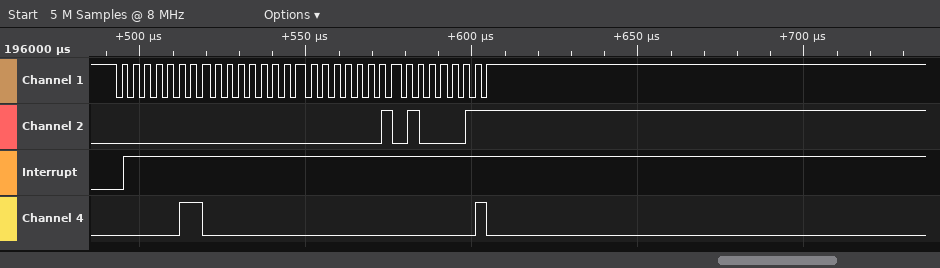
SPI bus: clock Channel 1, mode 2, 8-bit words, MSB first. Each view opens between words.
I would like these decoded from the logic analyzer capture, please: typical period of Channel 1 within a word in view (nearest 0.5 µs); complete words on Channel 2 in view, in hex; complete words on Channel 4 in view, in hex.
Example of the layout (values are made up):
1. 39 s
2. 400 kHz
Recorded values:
1. 3.5 µs
2. 00, 00, 01, 43
3. 03, 00, 00, 01
